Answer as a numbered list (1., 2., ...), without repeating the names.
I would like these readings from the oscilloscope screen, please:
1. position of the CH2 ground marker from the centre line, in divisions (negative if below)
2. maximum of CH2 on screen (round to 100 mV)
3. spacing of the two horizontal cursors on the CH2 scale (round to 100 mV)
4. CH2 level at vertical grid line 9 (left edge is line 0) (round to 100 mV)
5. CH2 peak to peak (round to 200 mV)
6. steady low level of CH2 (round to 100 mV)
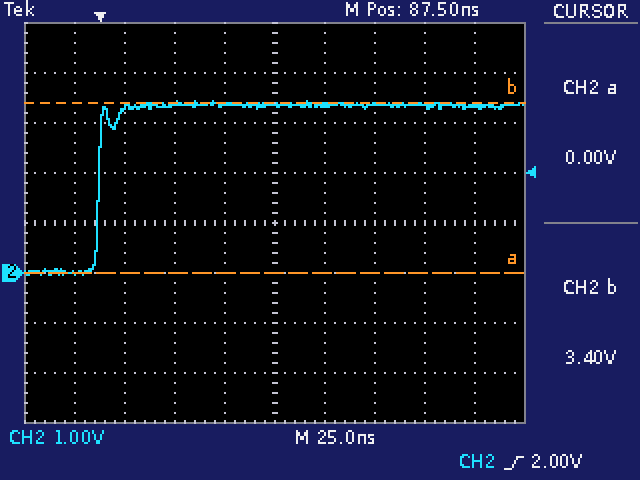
1. -1.0 div
2. 3.4 V
3. 3.4 V
4. 3.3 V
5. 3.4 V
6. 0.0 V
